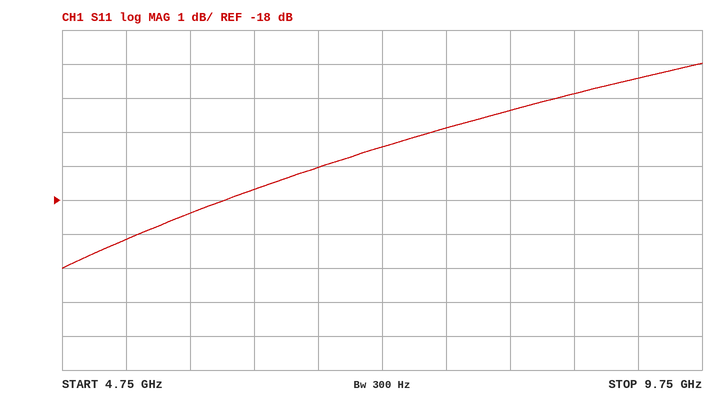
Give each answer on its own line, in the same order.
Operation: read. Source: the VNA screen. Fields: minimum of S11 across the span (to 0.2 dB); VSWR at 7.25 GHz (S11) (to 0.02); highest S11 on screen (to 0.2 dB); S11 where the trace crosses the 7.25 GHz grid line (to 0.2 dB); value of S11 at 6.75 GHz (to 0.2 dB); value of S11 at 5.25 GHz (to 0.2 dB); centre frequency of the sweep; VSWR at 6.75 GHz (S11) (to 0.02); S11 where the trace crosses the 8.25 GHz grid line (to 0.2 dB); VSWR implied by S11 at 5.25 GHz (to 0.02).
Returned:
-20.0 dB
1.36
-14.0 dB
-16.4 dB
-17.0 dB
-19.2 dB
7.25 GHz
1.32
-15.4 dB
1.24
